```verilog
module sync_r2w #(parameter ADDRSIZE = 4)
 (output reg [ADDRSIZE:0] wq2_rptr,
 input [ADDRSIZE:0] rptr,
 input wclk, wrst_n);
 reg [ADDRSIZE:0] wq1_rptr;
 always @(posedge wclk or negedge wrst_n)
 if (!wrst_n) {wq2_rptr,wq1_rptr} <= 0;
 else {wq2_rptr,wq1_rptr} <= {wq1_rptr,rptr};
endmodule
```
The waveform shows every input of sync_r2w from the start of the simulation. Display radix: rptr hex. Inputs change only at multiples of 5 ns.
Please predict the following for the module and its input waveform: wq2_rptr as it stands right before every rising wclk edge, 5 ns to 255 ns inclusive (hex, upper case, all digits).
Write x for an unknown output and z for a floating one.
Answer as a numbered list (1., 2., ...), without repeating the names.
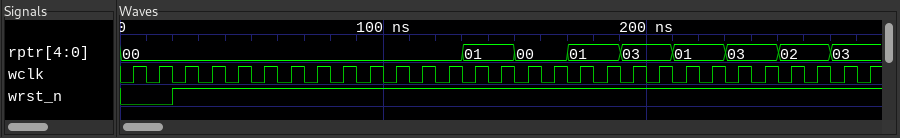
1. 00, 00, 00, 00, 00, 00, 00, 00, 00, 00, 00, 00, 00, 00, 00, 01, 01, 00, 00, 01, 01, 03, 03, 01, 01, 03
